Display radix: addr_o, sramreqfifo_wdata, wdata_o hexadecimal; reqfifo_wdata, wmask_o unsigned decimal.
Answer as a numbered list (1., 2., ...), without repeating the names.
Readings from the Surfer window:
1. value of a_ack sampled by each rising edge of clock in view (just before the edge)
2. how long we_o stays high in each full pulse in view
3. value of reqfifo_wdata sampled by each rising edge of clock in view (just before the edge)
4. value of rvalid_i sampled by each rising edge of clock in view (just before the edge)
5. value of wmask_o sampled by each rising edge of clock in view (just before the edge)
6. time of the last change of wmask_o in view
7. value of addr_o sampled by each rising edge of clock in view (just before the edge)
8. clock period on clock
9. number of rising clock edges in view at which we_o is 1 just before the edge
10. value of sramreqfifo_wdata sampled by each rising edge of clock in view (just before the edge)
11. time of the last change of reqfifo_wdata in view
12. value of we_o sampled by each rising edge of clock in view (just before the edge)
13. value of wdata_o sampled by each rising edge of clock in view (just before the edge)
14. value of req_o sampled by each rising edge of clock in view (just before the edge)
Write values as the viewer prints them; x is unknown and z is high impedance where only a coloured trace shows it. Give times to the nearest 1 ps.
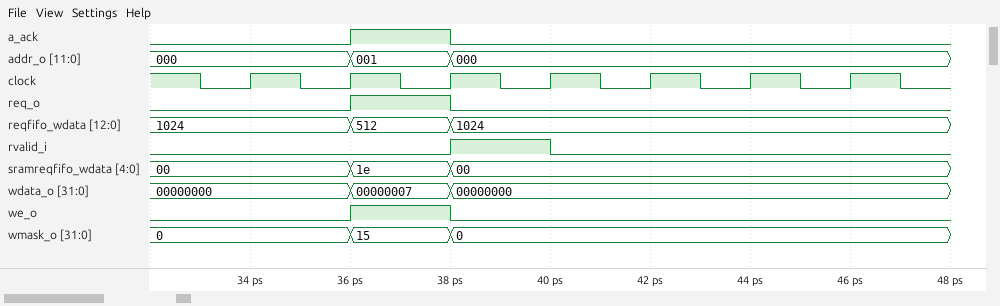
1. 0 0 1 0 0 0 0
2. 2 ps
3. 1024, 1024, 512, 1024, 1024, 1024, 1024
4. 0 0 0 1 0 0 0
5. 0, 0, 15, 0, 0, 0, 0
6. 38 ps
7. 000, 000, 001, 000, 000, 000, 000
8. 2 ps
9. 1
10. 00, 00, 1e, 00, 00, 00, 00
11. 38 ps
12. 0 0 1 0 0 0 0
13. 00000000, 00000000, 00000007, 00000000, 00000000, 00000000, 00000000
14. 0 0 1 0 0 0 0
